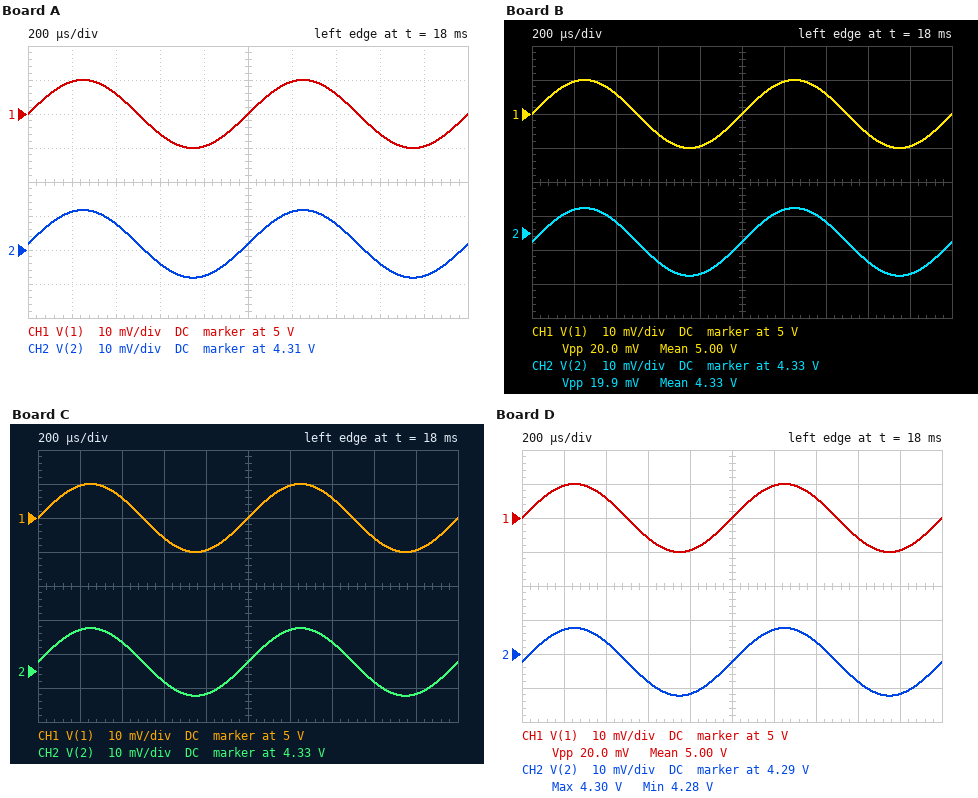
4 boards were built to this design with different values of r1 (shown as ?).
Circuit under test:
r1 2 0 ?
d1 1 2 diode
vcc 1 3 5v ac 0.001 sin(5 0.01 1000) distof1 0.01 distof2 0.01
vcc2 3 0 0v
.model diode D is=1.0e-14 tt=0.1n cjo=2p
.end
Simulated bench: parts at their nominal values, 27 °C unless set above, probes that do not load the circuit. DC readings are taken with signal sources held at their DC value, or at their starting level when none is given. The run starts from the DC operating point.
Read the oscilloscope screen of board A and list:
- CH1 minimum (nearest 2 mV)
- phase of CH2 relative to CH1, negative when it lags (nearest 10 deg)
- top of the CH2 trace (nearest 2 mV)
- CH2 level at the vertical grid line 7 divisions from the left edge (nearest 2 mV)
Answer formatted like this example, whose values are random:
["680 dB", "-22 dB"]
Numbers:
["4.990 V", "0 deg", "4.322 V", "4.318 V"]
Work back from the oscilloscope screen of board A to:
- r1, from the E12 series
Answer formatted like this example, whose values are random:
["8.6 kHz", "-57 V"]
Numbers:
["1.2 kΩ"]
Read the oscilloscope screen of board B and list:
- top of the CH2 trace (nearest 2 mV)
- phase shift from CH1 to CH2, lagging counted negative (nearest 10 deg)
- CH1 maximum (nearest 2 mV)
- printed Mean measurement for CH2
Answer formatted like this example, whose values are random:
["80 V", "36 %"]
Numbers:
["4.338 V", "0 deg", "5.010 V", "4.33 V"]
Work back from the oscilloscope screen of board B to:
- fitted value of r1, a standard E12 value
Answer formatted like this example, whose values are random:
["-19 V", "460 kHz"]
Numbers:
["2.2 kΩ"]
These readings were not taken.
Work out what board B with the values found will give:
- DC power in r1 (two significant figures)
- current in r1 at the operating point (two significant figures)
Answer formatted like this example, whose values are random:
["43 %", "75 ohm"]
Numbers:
["8.5 mW", "2.0 mA"]
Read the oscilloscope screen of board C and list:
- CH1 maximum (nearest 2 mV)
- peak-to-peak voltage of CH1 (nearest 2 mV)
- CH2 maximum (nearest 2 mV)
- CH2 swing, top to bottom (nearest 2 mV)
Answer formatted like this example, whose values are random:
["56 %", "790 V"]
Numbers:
["5.010 V", "20 mV", "4.342 V", "20 mV"]
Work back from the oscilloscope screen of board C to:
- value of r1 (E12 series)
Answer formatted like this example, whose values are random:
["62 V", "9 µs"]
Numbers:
["2.7 kΩ"]
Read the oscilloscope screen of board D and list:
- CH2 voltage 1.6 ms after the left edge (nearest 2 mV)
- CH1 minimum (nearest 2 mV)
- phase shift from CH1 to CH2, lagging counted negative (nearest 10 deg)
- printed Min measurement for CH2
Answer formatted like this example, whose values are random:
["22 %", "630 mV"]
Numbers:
["4.282 V", "4.990 V", "0 deg", "4.28 V"]
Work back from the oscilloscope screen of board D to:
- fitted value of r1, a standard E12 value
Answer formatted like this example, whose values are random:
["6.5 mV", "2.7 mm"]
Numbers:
["470 Ω"]
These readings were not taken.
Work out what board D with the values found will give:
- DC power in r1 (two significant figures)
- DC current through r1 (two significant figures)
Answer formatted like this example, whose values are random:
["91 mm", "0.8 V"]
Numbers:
["39 mW", "9.1 mA"]
